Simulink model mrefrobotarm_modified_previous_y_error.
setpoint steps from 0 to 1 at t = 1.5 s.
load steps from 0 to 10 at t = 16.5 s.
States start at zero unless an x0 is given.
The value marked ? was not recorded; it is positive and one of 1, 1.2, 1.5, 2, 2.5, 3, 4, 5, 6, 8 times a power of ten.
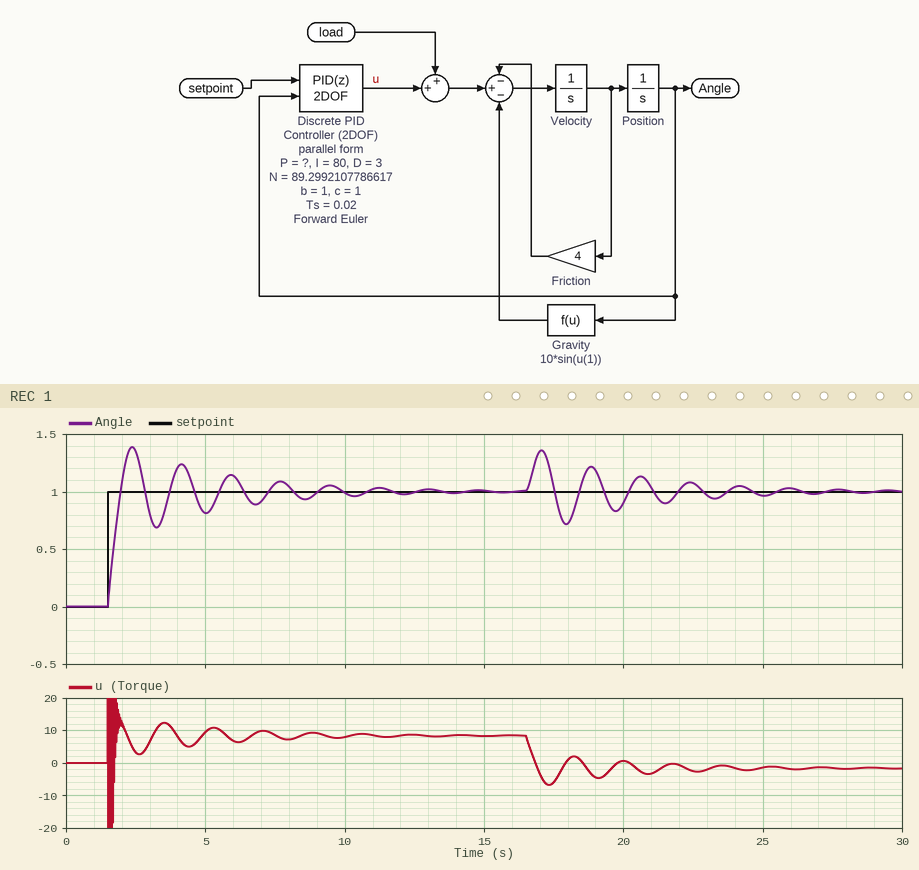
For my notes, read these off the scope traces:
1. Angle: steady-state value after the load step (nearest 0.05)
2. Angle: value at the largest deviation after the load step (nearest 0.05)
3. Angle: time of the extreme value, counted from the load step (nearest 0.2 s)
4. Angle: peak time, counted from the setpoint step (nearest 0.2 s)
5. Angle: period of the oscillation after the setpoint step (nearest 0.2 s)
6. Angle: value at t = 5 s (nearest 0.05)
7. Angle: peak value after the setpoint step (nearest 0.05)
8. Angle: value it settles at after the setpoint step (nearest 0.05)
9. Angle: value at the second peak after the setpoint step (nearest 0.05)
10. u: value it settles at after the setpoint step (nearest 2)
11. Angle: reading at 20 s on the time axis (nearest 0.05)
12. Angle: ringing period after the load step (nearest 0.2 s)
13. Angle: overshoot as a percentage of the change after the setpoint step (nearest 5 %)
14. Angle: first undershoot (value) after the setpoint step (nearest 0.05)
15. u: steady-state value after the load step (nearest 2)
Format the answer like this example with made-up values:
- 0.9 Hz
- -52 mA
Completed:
- 1.00
- 1.35
- 0.6 s
- 0.8 s
- 1.8 s
- 0.80
- 1.40
- 1.00
- 1.25
- 8
- 0.90
- 1.8 s
- 40 %
- 0.70
- -2
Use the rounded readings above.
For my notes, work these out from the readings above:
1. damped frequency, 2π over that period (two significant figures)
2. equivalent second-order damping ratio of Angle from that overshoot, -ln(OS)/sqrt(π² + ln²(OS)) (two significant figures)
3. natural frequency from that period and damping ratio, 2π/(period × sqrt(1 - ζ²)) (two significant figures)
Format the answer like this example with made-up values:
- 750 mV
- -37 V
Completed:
- 3.5 rad/s
- 0.28
- 3.6 rad/s
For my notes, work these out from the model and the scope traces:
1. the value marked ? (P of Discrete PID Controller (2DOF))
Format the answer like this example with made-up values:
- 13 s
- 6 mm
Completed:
- 12
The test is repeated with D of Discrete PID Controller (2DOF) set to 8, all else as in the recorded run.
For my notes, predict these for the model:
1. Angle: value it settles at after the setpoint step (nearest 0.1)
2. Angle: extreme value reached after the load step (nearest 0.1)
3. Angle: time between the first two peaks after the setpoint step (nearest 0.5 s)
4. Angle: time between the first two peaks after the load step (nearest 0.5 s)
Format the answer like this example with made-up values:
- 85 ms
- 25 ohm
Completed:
- 1.0
- 1.3
- 2.5 s
- 2.5 s
